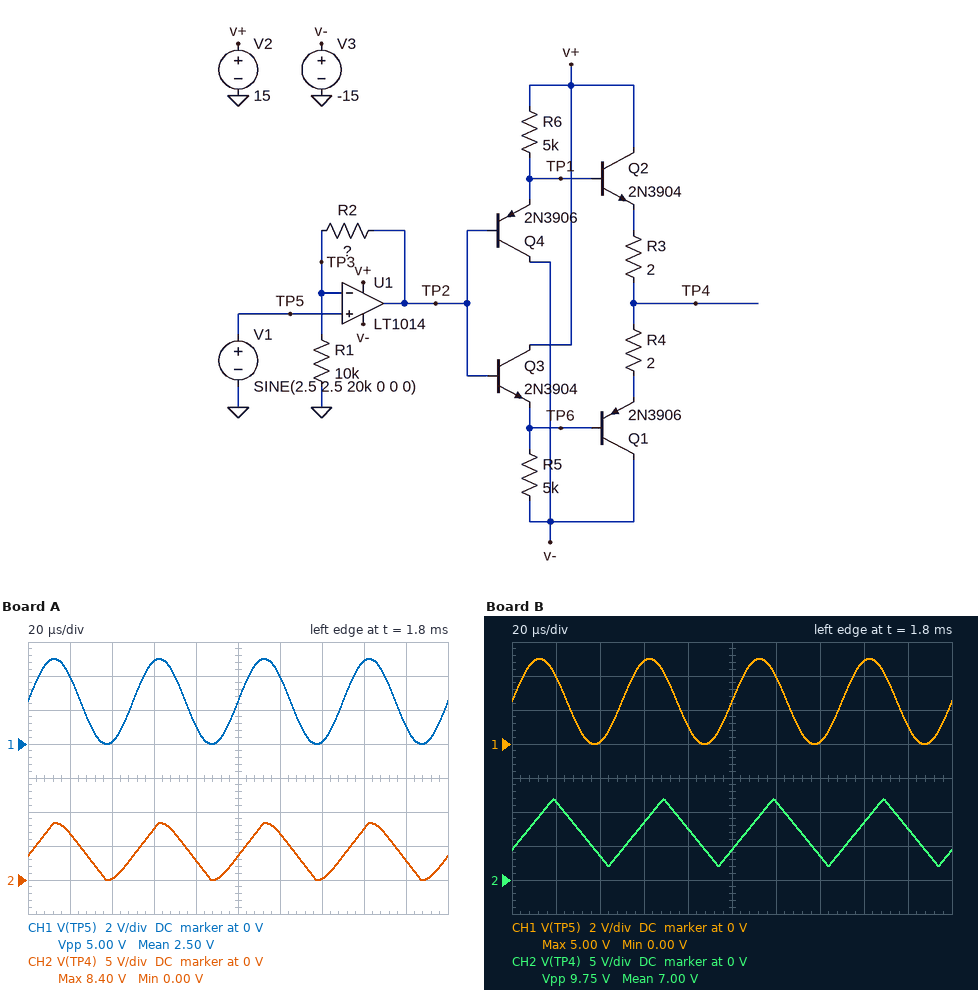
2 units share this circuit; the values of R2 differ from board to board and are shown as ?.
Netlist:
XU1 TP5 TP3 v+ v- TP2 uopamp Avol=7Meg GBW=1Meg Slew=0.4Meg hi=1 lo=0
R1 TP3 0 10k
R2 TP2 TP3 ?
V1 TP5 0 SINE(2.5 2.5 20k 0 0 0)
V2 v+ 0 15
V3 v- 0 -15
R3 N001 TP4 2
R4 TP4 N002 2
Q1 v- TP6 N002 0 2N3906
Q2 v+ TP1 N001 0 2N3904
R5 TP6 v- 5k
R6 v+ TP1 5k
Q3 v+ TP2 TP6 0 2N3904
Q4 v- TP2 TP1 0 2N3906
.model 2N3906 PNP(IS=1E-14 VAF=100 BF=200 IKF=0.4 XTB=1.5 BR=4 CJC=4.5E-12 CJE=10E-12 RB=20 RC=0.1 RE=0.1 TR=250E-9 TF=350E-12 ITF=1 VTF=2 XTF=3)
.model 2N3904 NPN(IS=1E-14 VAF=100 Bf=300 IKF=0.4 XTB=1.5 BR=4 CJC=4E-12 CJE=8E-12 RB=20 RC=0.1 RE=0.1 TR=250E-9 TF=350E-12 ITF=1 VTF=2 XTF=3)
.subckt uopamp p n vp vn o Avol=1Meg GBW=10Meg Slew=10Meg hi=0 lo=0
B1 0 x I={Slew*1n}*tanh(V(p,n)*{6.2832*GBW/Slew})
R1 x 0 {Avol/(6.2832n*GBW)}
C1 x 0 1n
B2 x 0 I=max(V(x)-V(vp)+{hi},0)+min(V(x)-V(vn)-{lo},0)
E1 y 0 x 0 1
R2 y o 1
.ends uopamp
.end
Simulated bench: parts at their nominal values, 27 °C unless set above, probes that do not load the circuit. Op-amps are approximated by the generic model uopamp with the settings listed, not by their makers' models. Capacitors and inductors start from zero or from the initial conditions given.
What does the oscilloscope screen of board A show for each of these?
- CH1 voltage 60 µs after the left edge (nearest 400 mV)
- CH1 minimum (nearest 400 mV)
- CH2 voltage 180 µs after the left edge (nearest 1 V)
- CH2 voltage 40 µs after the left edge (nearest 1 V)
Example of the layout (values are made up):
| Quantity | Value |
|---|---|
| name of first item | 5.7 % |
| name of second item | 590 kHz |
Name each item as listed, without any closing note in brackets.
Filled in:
| Quantity | Value |
|---|---|
| CH1 voltage 60 µs after the left edge | 4.8 V |
| CH1 minimum | 0 V |
| CH2 voltage 180 µs after the left edge | 3 V |
| CH2 voltage 40 µs after the left edge | 0 V |
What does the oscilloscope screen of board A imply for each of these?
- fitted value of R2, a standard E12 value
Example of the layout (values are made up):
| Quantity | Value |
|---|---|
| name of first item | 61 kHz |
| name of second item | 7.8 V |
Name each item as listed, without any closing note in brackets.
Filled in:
| Quantity | Value |
|---|---|
| fitted value of R2, a standard E12 value | 6.8 kΩ |
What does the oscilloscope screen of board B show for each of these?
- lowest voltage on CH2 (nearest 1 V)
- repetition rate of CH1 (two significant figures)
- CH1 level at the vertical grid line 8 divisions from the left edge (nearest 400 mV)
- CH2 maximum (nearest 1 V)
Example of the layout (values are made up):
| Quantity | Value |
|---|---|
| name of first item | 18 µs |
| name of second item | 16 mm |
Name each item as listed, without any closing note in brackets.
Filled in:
| Quantity | Value |
|---|---|
| lowest voltage on CH2 | 2 V |
| repetition rate of CH1 | 20 kHz |
| CH1 level at the vertical grid line 8 divisions from the left edge | 4.8 V |
| CH2 maximum | 12 V |
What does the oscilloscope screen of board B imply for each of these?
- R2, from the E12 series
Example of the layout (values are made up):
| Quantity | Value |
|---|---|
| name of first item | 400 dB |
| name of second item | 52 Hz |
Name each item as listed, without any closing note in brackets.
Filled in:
| Quantity | Value |
|---|---|
| R2, from the E12 series | 18 kΩ |
